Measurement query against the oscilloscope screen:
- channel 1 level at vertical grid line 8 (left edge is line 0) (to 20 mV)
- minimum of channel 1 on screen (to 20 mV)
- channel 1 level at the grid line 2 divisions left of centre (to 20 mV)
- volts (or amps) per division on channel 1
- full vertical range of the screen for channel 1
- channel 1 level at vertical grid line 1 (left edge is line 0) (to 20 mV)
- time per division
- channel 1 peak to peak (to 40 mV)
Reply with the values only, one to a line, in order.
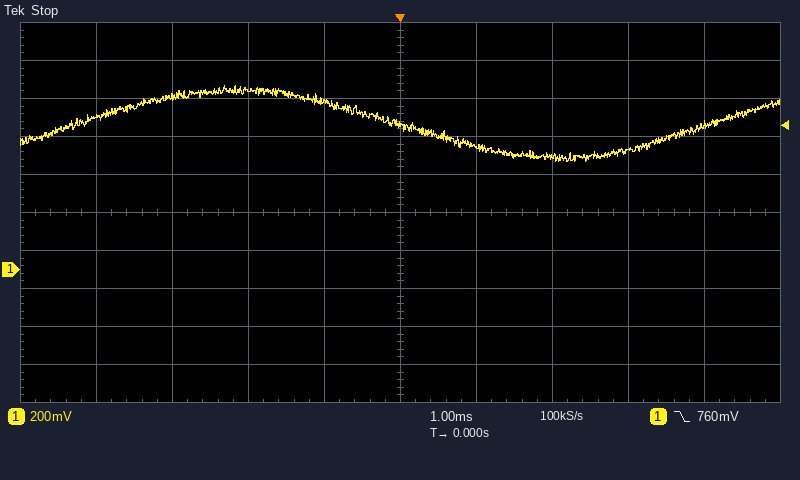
620 mV
560 mV
940 mV
200 mV
2 V
800 mV
1 ms
400 mV
